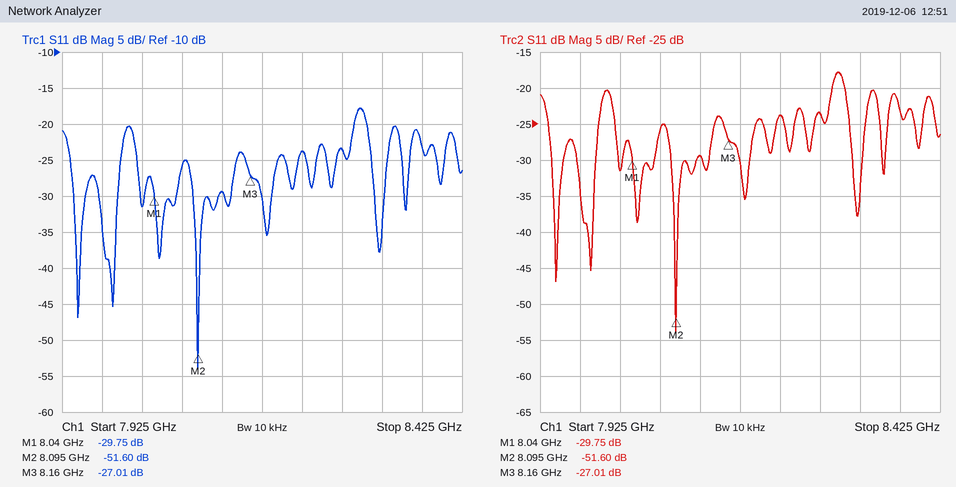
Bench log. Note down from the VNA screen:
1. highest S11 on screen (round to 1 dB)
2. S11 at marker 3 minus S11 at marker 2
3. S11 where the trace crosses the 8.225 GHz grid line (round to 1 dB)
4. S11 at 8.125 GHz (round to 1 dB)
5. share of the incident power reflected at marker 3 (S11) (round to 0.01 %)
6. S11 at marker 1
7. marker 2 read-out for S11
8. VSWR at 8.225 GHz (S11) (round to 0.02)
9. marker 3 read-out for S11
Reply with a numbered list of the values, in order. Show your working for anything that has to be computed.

1. -18 dB
2. -27.01 − (-51.6) = 24.59 dB
3. -24 dB
4. -29 dB
5. 10^(-27.01/10) ≈ 0.20 %
6. -29.75 dB
7. -51.60 dB
8. |Γ| = 10^(-24/20) = 0.0631; VSWR = (1 + 0.0631)/(1 − 0.0631) ≈ 1.13, so 1.14 to the nearest 0.02
9. -27.01 dB
